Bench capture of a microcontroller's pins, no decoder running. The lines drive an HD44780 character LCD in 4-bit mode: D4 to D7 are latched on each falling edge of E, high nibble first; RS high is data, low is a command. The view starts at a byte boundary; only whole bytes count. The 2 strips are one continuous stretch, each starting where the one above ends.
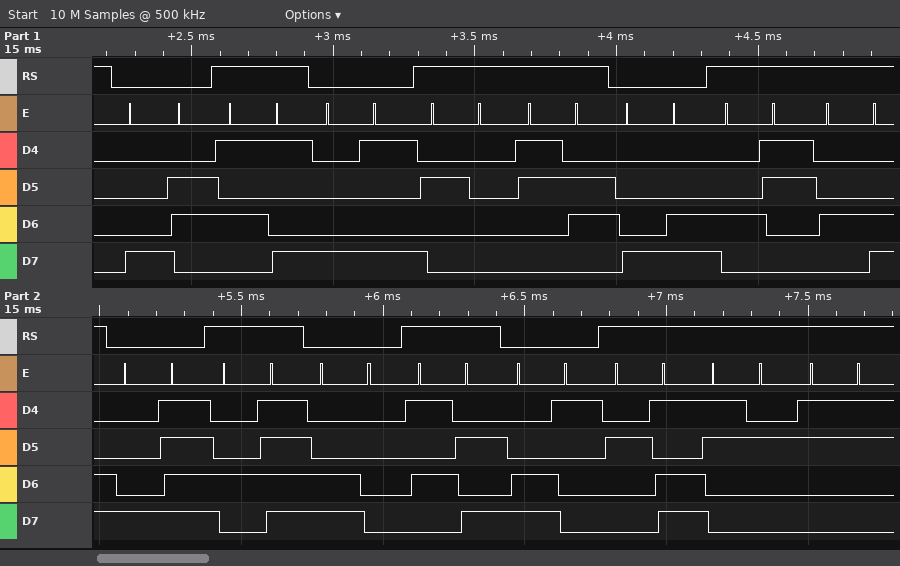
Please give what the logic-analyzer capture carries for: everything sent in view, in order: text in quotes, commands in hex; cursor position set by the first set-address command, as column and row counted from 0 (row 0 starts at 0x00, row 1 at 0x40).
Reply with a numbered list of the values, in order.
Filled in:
1. 0x86 "Y" 0x89 " 6" 0x8C "CL" 0x8F "O" 0xC0 "Z" 0xC1 "-23"
2. column 6, row 0
